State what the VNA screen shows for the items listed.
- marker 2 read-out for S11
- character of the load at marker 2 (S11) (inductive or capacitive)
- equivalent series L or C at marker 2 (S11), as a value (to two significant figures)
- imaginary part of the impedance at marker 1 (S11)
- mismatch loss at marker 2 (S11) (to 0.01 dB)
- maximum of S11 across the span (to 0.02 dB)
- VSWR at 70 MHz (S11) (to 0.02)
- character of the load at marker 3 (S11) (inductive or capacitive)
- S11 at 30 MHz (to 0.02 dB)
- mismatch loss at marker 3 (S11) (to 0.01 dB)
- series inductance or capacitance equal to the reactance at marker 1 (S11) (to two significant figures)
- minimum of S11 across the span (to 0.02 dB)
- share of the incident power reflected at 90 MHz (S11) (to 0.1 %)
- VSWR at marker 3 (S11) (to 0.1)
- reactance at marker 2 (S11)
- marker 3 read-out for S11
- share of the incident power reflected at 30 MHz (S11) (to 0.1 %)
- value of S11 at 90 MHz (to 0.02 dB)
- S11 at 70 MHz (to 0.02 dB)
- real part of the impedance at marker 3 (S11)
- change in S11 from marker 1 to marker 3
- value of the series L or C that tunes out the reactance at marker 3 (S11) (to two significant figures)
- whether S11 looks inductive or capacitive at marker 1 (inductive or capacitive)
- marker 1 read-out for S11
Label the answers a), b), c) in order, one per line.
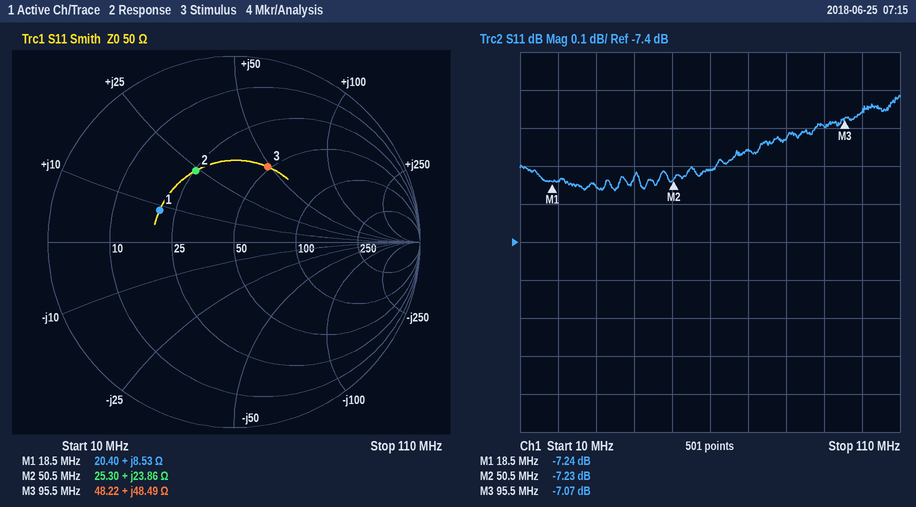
a) -7.23 dB
b) inductive
c) 75 nH
d) +8.53 Ω
e) 0.91 dB
f) -7.02 dB
g) 2.56
h) inductive
i) -7.26 dB
j) 0.95 dB
k) 73 nH
l) -7.26 dB
m) 19.5 %
n) 2.6
o) +23.86 Ω
p) -7.07 dB
q) 18.8 %
r) -7.10 dB
s) -7.16 dB
t) 48.22 Ω
u) 0.17 dB
v) 34 pF
w) inductive
x) -7.24 dB
